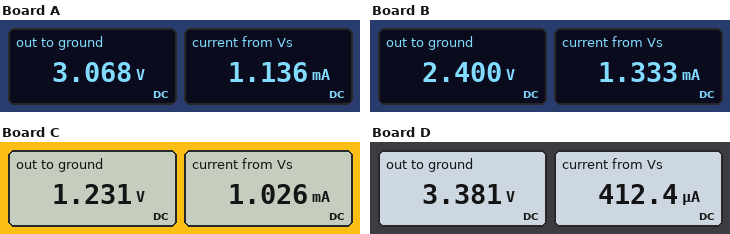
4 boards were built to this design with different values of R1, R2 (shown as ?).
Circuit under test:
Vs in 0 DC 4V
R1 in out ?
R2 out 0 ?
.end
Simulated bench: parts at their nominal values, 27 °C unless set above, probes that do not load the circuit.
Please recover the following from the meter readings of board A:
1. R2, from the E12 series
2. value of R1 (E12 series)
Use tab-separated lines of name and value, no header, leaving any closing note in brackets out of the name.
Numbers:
R2, from the E12 series	2.7 kΩ
value of R1	820 Ω
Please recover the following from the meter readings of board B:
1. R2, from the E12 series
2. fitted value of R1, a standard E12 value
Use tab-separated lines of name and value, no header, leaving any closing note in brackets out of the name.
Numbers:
R2, from the E12 series	1.8 kΩ
fitted value of R1, a standard E12 value	1.2 kΩ
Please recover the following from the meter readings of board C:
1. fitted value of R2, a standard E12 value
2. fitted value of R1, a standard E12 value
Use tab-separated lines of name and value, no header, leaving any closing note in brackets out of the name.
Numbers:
fitted value of R2, a standard E12 value	1.2 kΩ
fitted value of R1, a standard E12 value	2.7 kΩ
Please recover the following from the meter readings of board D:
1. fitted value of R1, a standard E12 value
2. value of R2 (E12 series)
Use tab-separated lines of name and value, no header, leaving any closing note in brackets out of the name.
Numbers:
fitted value of R1, a standard E12 value	1.5 kΩ
value of R2	8.2 kΩ
